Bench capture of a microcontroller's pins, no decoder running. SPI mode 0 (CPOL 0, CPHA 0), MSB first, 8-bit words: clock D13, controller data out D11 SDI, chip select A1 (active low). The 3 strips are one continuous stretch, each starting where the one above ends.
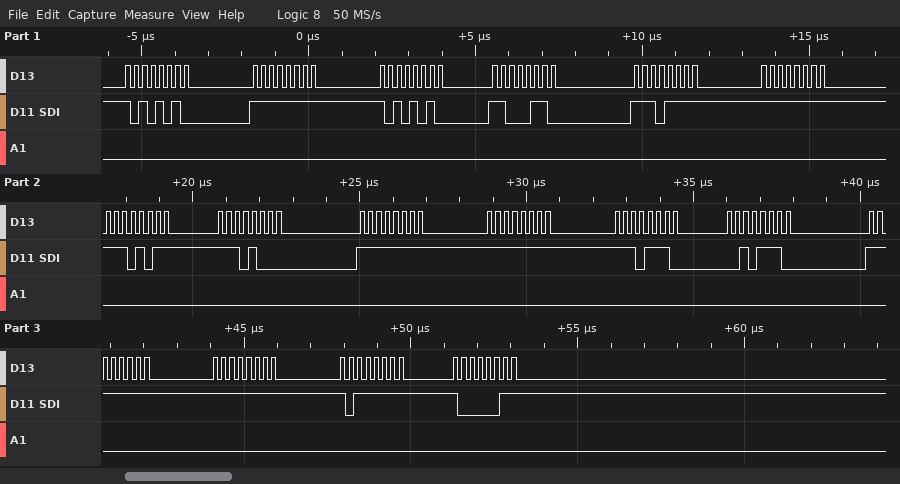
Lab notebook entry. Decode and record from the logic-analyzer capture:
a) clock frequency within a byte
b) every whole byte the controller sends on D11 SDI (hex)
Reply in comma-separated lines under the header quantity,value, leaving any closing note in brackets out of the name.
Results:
quantity,value
clock frequency within a byte,4 MHz
every whole byte the controller sends on D11 SDI,0xAA 0xFF 0xAA 0xC6 0xEF 0xFF 0xEB 0xE8 0xFF 0xFF 0xEE 0x2E 0xFF 0xFF 0xBF 0x83
